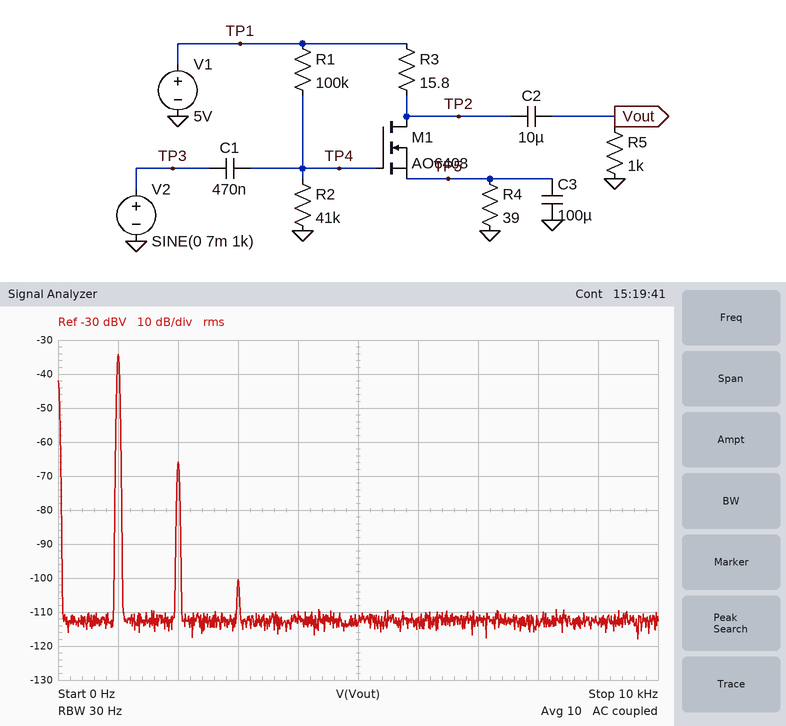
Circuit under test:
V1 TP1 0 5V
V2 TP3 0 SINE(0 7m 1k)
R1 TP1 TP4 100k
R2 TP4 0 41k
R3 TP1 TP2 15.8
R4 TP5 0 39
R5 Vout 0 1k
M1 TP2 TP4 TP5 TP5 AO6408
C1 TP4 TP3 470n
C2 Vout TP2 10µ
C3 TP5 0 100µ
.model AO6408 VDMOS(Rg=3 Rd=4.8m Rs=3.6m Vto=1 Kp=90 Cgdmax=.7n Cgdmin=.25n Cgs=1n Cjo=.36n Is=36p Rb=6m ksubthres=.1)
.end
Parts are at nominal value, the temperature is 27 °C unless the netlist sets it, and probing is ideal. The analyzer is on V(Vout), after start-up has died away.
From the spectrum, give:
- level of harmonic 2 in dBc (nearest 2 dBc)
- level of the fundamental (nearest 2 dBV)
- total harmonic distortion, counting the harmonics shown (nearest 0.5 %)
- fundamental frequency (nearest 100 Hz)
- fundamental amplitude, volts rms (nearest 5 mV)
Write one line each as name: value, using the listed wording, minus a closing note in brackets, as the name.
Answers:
level of harmonic 2 in dBc: -32 dBc
level of the fundamental: -34 dBV
total harmonic distortion, counting the harmonics shown: 2.5 %
fundamental frequency: 1.0 kHz
fundamental amplitude, volts rms: 20 mV
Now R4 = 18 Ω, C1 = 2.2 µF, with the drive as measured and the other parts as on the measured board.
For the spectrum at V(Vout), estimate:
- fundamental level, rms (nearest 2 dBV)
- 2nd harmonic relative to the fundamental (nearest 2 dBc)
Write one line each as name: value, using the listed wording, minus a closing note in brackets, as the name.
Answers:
fundamental level, rms: -30 dBV
2nd harmonic relative to the fundamental: -34 dBc
